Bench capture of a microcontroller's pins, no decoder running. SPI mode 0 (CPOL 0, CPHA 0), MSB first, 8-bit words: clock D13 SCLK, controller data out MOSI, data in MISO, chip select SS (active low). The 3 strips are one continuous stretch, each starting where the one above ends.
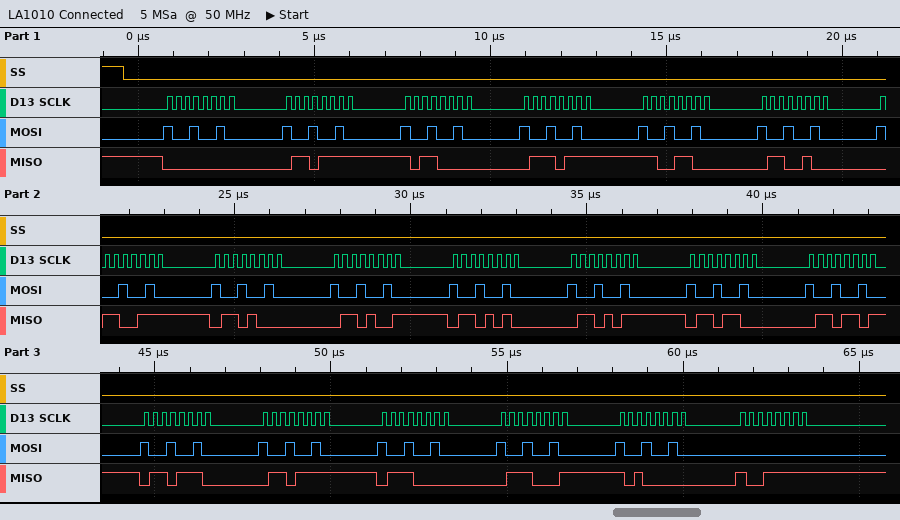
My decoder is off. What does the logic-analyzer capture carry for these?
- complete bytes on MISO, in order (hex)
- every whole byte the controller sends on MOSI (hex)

00 6F B0 77 CC 64 67 68 69 6A 6B 6C 6D 6E 6F 70 71 A0 9F
92 92 92 92 92 92 92 92 92 92 92 92 92 92 92 92 92 92 00
